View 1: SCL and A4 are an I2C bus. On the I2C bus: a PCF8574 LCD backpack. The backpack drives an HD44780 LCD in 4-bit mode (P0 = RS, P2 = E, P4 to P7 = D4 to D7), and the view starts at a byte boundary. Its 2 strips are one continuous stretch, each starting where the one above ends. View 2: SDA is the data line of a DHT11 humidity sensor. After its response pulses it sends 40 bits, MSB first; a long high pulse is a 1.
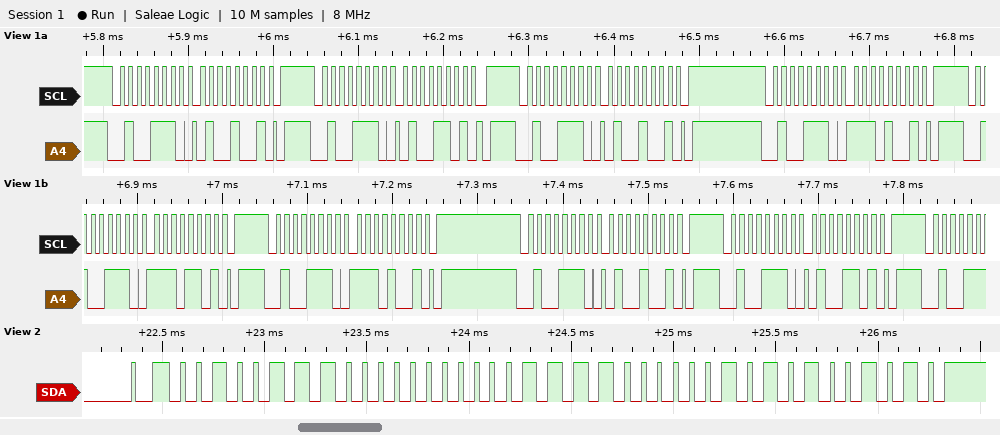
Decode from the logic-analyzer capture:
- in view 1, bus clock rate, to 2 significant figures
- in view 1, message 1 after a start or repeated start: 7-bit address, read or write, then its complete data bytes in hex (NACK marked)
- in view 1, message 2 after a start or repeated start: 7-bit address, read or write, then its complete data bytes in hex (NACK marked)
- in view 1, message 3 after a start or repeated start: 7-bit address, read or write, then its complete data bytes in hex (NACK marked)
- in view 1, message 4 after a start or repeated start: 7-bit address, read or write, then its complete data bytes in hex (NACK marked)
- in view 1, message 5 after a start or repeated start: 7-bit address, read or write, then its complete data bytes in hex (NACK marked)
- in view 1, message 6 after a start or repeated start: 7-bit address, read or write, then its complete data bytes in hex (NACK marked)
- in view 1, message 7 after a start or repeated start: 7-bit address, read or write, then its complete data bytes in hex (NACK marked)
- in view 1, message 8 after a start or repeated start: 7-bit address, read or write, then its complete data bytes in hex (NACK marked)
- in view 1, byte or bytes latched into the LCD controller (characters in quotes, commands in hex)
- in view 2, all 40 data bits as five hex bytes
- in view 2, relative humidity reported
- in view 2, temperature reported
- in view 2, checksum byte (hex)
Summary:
100 kHz
0x27 write: 49
0x27 write: 4D
0x27 write: 49
0x27 write: E9
0x27 write: ED
0x27 write: E9
0x27 write: 49
0x27 write: 4D
'N'
27 00 1E 05 4A
39 %
30.5 °C
0x4A
